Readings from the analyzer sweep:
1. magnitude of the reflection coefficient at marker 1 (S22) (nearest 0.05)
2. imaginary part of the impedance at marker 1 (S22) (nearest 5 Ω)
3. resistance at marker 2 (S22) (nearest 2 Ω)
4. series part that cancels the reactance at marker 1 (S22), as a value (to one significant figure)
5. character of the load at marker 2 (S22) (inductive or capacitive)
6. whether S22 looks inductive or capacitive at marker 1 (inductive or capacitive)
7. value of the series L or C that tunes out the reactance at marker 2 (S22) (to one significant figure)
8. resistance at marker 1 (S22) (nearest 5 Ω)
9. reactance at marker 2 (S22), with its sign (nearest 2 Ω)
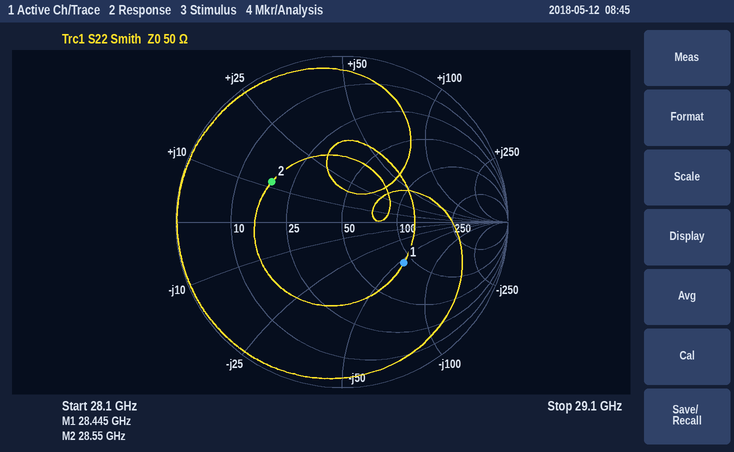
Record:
0.45
-55 Ω
18 Ω
300 pH
inductive
capacitive
500 fF
90 Ω
+12 Ω
